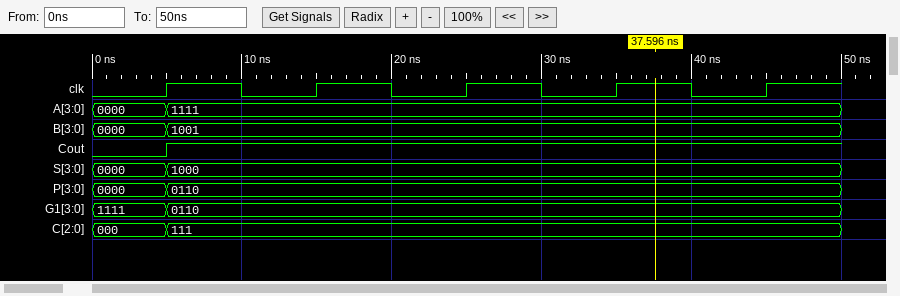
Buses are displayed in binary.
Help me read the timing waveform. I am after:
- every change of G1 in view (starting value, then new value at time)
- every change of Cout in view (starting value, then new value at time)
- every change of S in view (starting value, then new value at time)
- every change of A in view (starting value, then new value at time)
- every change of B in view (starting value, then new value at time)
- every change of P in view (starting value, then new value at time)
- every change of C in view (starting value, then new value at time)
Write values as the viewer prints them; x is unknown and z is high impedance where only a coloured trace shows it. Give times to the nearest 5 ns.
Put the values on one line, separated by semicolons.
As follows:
1111, 0110 at 5 ns; 0, 1 at 5 ns; 0000, 1000 at 5 ns; 0000, 1111 at 5 ns; 0000, 1001 at 5 ns; 0000, 0110 at 5 ns; 000, 111 at 5 ns
